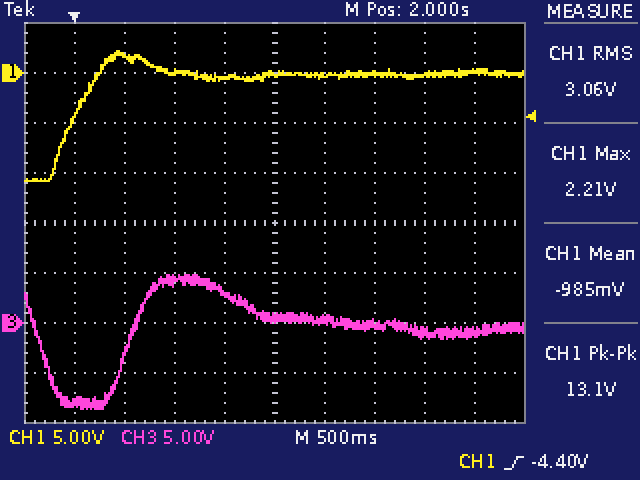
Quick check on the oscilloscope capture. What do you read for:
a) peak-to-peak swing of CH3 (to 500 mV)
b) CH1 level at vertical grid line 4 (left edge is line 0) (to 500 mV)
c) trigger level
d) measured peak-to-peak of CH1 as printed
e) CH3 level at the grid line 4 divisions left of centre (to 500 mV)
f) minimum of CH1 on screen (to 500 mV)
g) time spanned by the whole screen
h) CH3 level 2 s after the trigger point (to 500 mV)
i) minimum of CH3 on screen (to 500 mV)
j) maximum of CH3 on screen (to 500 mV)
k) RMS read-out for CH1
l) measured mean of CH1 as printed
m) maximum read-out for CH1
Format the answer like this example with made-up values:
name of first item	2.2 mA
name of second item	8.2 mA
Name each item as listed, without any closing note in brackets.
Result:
peak-to-peak swing of CH3	13.5 V
CH1 level at vertical grid line 4 (left edge is line 0)	-500 mV
trigger level	-4.40 V
measured peak-to-peak of CH1 as printed	13.1 V
CH3 level at the grid line 4 divisions left of centre	-8.0 V
minimum of CH1 on screen	-11.0 V
time spanned by the whole screen	5 s
CH3 level 2 s after the trigger point	500 mV
minimum of CH3 on screen	-8.5 V
maximum of CH3 on screen	5.0 V
RMS read-out for CH1	3.06 V
measured mean of CH1 as printed	-985 mV
maximum read-out for CH1	2.21 V
